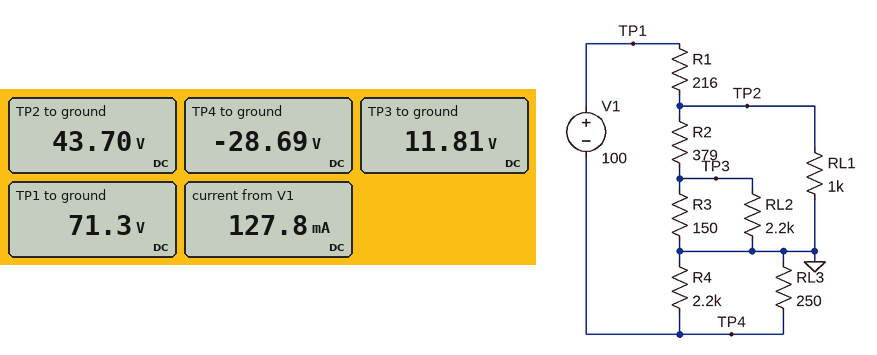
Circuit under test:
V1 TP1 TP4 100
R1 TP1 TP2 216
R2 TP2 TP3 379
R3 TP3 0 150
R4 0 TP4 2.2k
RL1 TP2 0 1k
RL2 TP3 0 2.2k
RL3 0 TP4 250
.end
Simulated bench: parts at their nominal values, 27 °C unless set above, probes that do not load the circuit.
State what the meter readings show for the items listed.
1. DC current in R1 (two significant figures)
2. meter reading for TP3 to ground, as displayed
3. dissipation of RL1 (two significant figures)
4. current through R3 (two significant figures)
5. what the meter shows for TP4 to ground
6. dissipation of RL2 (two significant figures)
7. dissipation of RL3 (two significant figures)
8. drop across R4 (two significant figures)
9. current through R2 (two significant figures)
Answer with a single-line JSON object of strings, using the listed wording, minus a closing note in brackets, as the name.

{"DC current in R1": "130 mA", "meter reading for TP3 to ground, as displayed": "11.81 V", "dissipation of RL1": "1.9 W", "current through R3": "79 mA", "what the meter shows for TP4 to ground": "-28.69 V", "dissipation of RL2": "63 mW", "dissipation of RL3": "3.3 W", "drop across R4": "29 V", "current through R2": "84 mA"}
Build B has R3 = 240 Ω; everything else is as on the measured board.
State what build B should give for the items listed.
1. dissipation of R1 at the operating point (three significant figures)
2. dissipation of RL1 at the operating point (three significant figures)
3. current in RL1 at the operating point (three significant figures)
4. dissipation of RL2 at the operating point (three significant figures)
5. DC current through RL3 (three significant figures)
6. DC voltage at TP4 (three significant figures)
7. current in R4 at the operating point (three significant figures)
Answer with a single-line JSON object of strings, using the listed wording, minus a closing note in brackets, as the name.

{"dissipation of R1 at the operating point": "3.26 W", "dissipation of RL1 at the operating point": "2.10 W", "current in RL1 at the operating point": "45.9 mA", "dissipation of RL2 at the operating point": "126 mW", "DC current through RL3": "110 mA", "DC voltage at TP4": "-27.6 V", "current in R4 at the operating point": "12.5 mA"}
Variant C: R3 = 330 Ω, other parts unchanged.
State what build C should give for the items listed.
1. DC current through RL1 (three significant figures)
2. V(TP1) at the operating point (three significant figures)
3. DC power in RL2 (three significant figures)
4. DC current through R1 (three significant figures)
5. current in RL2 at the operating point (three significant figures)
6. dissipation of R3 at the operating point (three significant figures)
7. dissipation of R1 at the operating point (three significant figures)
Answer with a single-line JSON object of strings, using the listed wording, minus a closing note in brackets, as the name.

{"DC current through RL1": "47.6 mA", "V(TP1) at the operating point": "73.3 V", "DC power in RL2": "191 mW", "DC current through R1": "119 mA", "current in RL2 at the operating point": "9.32 mA", "dissipation of R3 at the operating point": "1.27 W", "dissipation of R1 at the operating point": "3.06 W"}
